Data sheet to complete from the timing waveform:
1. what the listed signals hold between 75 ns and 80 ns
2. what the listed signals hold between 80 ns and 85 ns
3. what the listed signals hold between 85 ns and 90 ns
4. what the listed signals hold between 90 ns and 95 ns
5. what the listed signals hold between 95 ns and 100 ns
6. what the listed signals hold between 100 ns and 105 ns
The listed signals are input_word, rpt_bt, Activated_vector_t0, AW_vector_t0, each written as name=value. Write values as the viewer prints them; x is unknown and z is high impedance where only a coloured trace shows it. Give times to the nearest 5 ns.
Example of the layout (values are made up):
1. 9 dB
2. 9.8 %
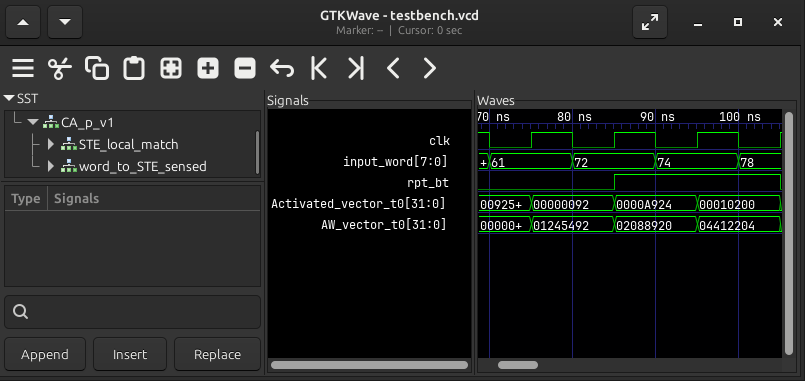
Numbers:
1. input_word=61, rpt_bt=0, Activated_vector_t0=00000092, AW_vector_t0=01245492
2. input_word=72, rpt_bt=0, Activated_vector_t0=00000092, AW_vector_t0=01245492
3. input_word=72, rpt_bt=1, Activated_vector_t0=0000A924, AW_vector_t0=02088920
4. input_word=74, rpt_bt=1, Activated_vector_t0=0000A924, AW_vector_t0=02088920
5. input_word=74, rpt_bt=1, Activated_vector_t0=00010200, AW_vector_t0=04412204
6. input_word=78, rpt_bt=1, Activated_vector_t0=00010200, AW_vector_t0=04412204
